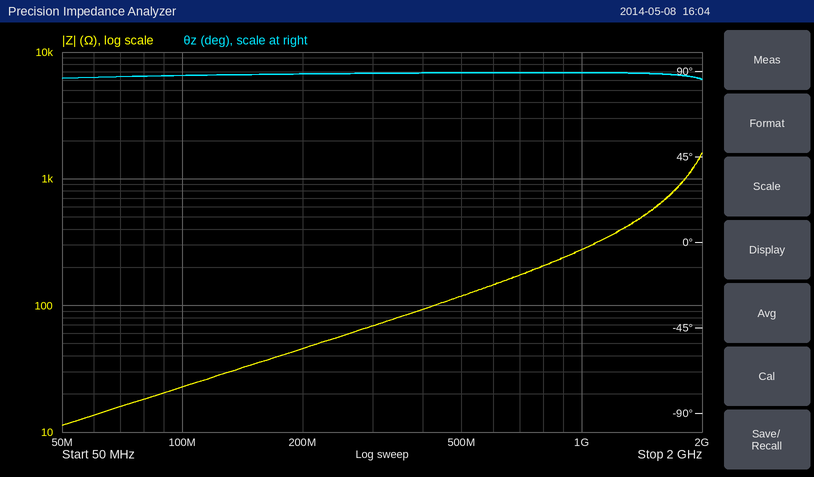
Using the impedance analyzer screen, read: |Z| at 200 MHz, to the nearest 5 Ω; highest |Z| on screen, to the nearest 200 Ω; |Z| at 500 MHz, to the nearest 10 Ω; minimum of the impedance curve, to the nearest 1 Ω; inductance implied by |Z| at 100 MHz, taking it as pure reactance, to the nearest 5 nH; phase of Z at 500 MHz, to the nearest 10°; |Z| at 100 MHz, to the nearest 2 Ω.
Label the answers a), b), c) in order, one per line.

a) 45 Ω
b) 1.6 kΩ
c) 120 Ω
d) 11 Ω
e) 35 nH
f) 90°
g) 22 Ω
